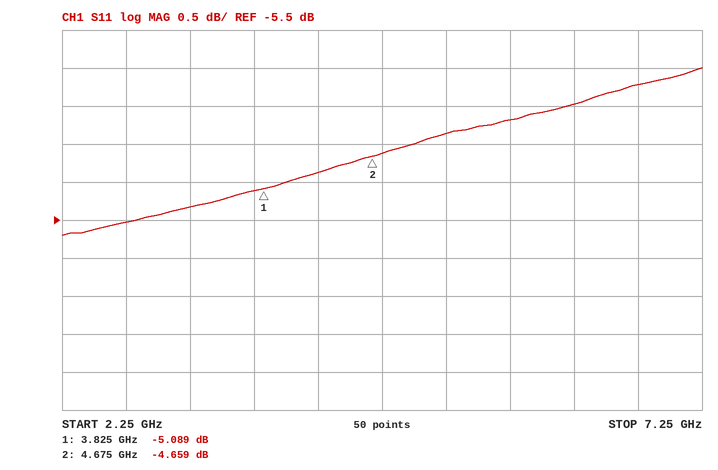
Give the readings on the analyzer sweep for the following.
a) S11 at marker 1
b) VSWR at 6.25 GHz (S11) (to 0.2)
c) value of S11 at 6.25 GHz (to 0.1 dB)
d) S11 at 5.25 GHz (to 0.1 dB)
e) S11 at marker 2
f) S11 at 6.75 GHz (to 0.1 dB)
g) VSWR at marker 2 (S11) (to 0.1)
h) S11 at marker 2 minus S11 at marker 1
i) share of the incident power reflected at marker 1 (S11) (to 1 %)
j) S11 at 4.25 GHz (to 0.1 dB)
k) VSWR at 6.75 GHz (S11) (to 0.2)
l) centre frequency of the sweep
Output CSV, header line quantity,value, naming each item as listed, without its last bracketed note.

quantity,value
S11 at marker 1,-5.089 dB
VSWR at 6.25 GHz (S11),4.4
value of S11 at 6.25 GHz,-4.0 dB
S11 at 5.25 GHz,-4.4 dB
S11 at marker 2,-4.659 dB
S11 at 6.75 GHz,-3.7 dB
VSWR at marker 2 (S11),3.8
S11 at marker 2 minus S11 at marker 1,0.430 dB
share of the incident power reflected at marker 1 (S11),31 %
S11 at 4.25 GHz,-4.9 dB
VSWR at 6.75 GHz (S11),4.8
centre frequency of the sweep,4.75 GHz
